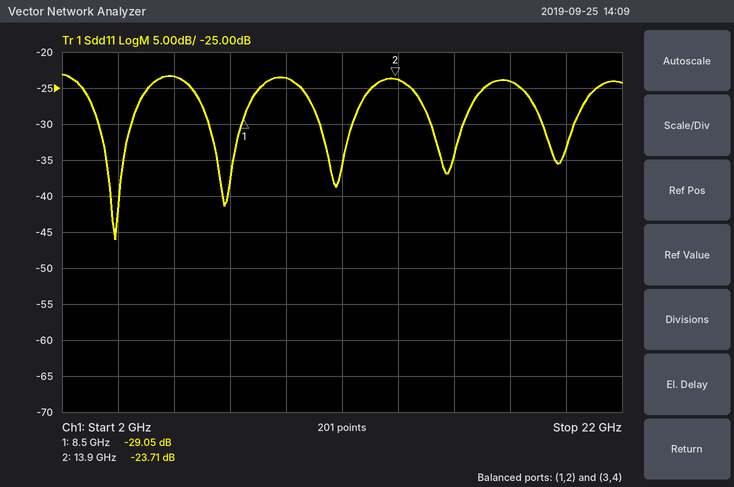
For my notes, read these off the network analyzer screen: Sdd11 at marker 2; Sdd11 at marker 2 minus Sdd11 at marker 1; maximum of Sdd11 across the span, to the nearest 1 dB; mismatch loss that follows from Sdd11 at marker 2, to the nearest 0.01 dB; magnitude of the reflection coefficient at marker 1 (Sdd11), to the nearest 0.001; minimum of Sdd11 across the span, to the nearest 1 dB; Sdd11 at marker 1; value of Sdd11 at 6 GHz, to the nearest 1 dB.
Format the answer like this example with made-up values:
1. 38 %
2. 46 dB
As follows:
1. -23.71 dB
2. 5.34 dB
3. -23 dB
4. 0.02 dB
5. 0.035
6. -46 dB
7. -29.05 dB
8. -23 dB
